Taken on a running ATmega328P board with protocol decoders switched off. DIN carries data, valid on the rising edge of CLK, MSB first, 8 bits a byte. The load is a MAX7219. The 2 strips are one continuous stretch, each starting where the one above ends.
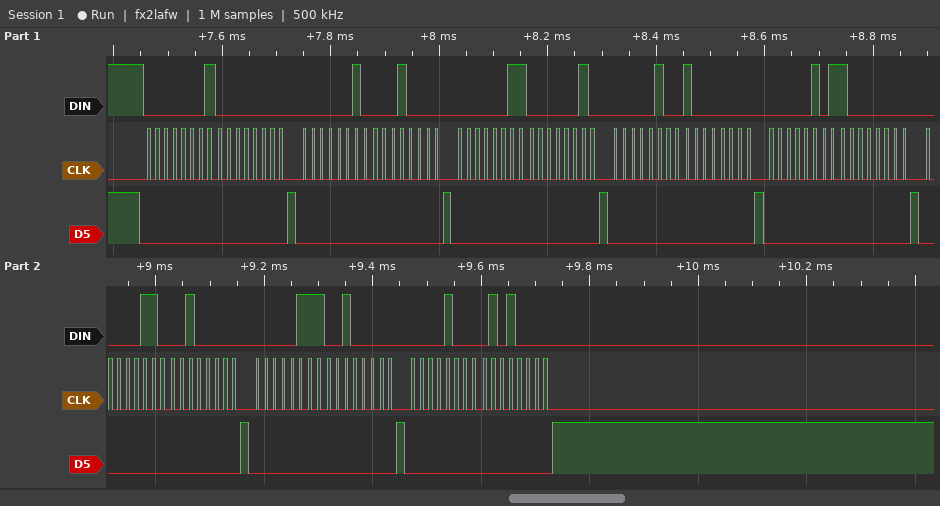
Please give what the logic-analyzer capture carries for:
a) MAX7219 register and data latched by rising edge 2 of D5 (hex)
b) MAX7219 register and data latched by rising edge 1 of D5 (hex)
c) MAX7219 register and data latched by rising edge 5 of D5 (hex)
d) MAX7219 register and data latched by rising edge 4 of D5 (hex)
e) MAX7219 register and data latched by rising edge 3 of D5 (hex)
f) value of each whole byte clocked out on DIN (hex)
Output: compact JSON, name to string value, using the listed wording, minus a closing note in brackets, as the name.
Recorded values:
{"MAX7219 register and data latched by rising edge 2 of D5": "register 0x2, data 0x10", "MAX7219 register and data latched by rising edge 1 of D5": "register 0x1, data 0x00", "MAX7219 register and data latched by rising edge 5 of D5": "register 0x5, data 0x80", "MAX7219 register and data latched by rising edge 4 of D5": "register 0x4, data 0x80", "MAX7219 register and data latched by rising edge 3 of D5": "register 0x3, data 0x02", "value of each whole byte clocked out on DIN": "01 00 02 10 03 02 04 80 05 80 06 20 07 20 08 50"}
